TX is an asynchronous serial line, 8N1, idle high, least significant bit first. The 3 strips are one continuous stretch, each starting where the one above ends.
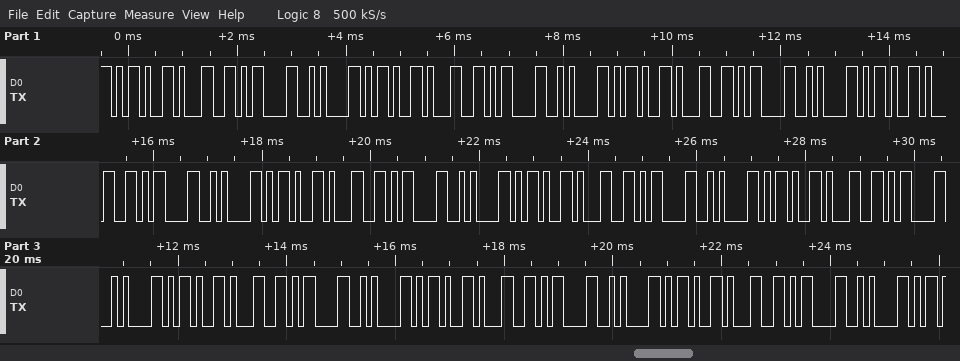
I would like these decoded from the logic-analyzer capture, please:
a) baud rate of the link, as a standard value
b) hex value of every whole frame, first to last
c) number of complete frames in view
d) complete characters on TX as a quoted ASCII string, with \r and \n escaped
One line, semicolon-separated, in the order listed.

9600 baud; 2D 31 0D 0A 2D 31 0D 0A 2D 31 0D 0A 2D 31 0D 0A 2D 31 0D 0A 2D 31 0D 0A 2D 31 0D 0A 2D 31 0D 0A 2D 31 0D 0A 2D 31 0D 0A; 40; "-1\r\n-1\r\n-1\r\n-1\r\n-1\r\n-1\r\n-1\r\n-1\r\n-1\r\n-1\r\n"
